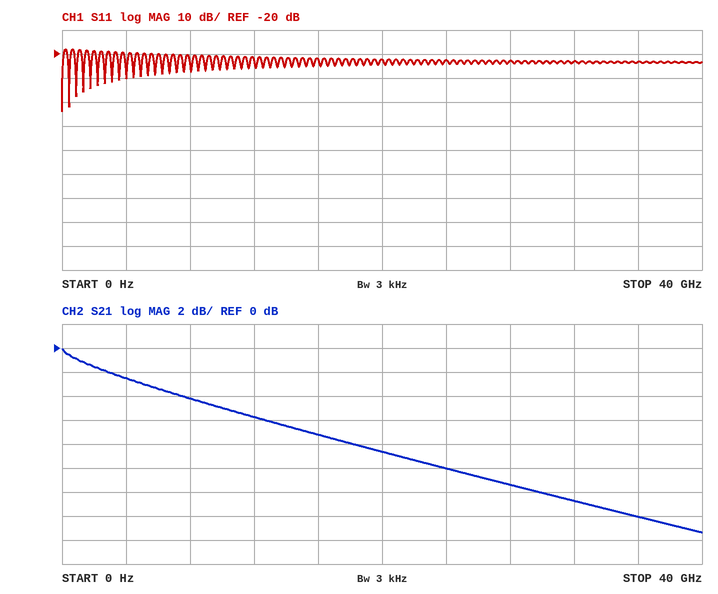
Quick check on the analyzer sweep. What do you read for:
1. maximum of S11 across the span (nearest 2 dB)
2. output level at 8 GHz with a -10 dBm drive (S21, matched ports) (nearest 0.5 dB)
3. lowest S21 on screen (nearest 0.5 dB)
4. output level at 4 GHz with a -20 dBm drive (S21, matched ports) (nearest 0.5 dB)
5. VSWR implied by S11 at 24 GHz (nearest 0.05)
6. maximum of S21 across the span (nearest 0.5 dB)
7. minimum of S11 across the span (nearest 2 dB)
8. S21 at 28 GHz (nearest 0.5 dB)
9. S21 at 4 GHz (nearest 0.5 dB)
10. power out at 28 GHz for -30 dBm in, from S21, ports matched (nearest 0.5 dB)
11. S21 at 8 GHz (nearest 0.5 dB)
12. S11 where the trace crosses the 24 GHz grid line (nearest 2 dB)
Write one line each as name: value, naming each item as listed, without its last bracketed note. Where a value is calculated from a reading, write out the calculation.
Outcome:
maximum of S11 across the span: -18 dB
output level at 8 GHz with a -10 dBm drive (S21, matched ports): -10 dBm + (-4.0 dB) = -14.0 dBm
lowest S21 on screen: -15.5 dB
output level at 4 GHz with a -20 dBm drive (S21, matched ports): -20 dBm + (-2.5 dB) = -22.5 dBm
VSWR implied by S11 at 24 GHz: |Γ| = 10^(-22/20) = 0.0794; VSWR = (1 + 0.0794)/(1 − 0.0794) ≈ 1.17, so 1.15 to the nearest 0.05
maximum of S21 across the span: 0.0 dB
minimum of S11 across the span: -44 dB
S21 at 28 GHz: -11.5 dB
S21 at 4 GHz: -2.5 dB
power out at 28 GHz for -30 dBm in, from S21, ports matched: -30 dBm + (-11.5 dB) = -41.5 dBm
S21 at 8 GHz: -4.0 dB
S11 where the trace crosses the 24 GHz grid line: -22 dB
